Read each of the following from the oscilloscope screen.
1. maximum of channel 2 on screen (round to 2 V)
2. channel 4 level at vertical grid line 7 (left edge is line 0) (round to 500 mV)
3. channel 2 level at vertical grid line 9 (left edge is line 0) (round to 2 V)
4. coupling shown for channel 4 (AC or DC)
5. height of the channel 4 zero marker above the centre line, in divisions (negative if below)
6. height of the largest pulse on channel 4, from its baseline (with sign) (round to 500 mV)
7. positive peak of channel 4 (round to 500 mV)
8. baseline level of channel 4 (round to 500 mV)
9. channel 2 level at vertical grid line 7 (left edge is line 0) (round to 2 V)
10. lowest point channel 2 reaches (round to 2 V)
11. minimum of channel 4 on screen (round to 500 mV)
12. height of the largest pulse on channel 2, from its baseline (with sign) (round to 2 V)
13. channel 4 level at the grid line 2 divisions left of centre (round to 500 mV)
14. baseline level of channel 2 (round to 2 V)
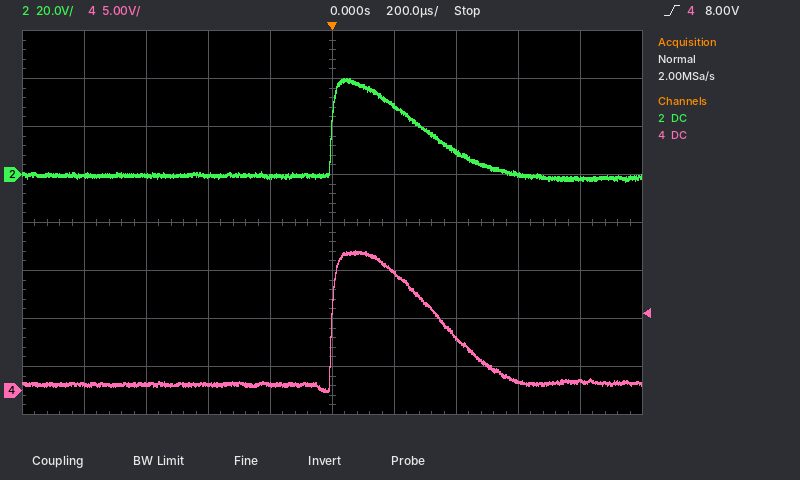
40 V
5.5 V
-2 V
DC
-3.5 div
+14.0 V
14.5 V
500 mV
10 V
-2 V
0.0 V
+40 V
500 mV
0 V
